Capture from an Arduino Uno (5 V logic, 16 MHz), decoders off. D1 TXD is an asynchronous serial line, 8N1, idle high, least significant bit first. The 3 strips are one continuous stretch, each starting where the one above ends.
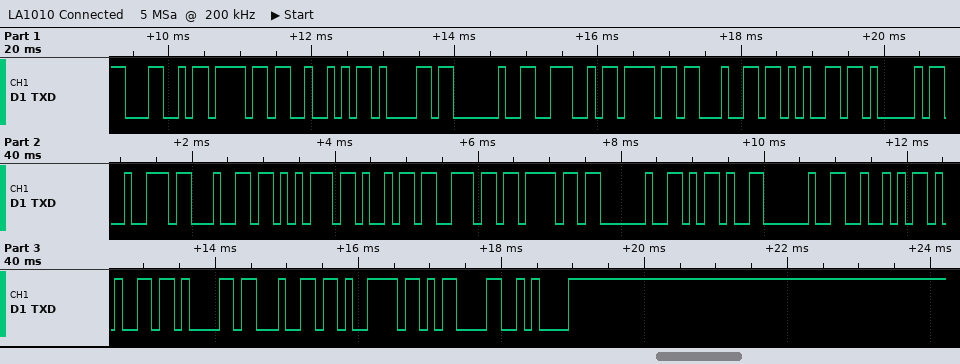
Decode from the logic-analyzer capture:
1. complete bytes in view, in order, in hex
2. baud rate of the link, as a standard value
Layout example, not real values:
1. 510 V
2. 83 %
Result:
1. 4C 6F 52 61 20 4E 6F 64 65 41 72 64 75 69 6E 6F 20 2D 20 52 65 61 64 79 0D 0A
2. 9600 baud
